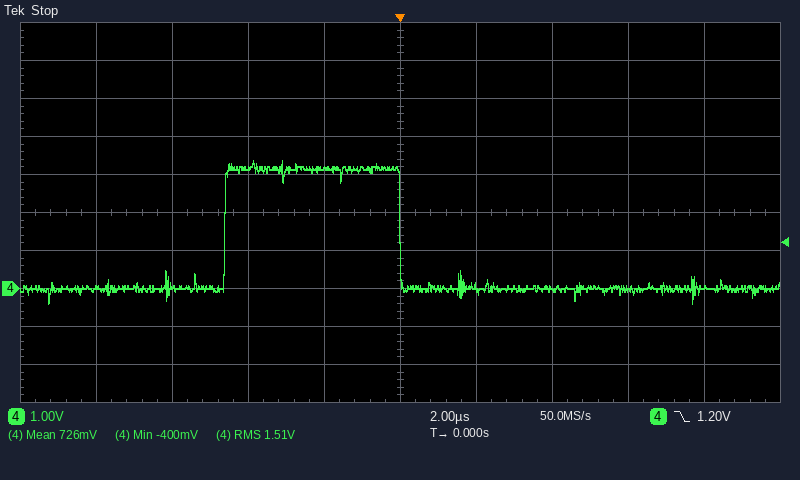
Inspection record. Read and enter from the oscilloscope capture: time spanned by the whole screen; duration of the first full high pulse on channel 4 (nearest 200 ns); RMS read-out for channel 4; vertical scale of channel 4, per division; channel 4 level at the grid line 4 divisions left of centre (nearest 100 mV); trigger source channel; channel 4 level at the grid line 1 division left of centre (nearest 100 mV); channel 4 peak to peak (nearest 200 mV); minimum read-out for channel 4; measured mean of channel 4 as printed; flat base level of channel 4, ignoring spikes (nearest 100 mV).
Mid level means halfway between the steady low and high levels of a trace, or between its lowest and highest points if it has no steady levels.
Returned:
20 µs
4.6 µs
1.51 V
1 V
0.0 V
channel 4
3.2 V
3.8 V
-400 mV
726 mV
0.0 V
